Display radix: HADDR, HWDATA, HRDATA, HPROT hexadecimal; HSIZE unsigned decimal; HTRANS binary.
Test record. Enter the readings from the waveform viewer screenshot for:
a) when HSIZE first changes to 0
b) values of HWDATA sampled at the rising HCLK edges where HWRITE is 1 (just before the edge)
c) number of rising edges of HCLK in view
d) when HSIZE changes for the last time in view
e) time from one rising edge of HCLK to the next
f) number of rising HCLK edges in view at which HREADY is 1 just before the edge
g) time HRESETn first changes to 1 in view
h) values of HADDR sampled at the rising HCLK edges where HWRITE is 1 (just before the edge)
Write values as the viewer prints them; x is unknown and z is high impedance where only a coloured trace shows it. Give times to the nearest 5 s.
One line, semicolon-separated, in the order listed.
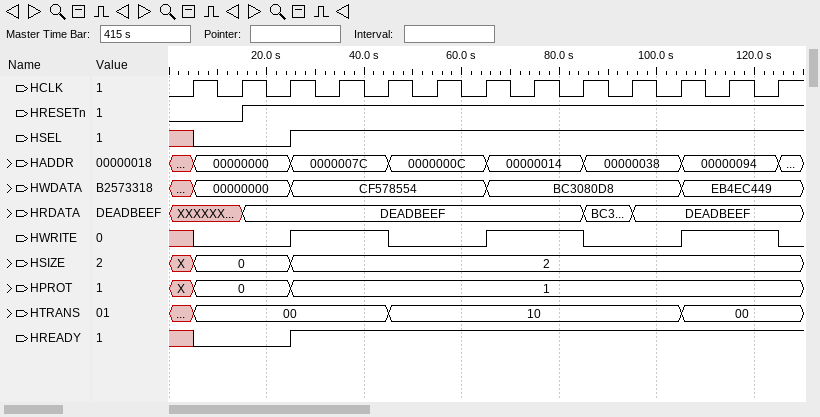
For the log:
5 s; CF578554, CF578554, BC3080D8, BC3080D8, EB4EC449, EB4EC449; 13; 25 s; 10 s; 10; 15 s; 0000007C, 0000007C, 00000014, 00000014, 00000094, 00000094
